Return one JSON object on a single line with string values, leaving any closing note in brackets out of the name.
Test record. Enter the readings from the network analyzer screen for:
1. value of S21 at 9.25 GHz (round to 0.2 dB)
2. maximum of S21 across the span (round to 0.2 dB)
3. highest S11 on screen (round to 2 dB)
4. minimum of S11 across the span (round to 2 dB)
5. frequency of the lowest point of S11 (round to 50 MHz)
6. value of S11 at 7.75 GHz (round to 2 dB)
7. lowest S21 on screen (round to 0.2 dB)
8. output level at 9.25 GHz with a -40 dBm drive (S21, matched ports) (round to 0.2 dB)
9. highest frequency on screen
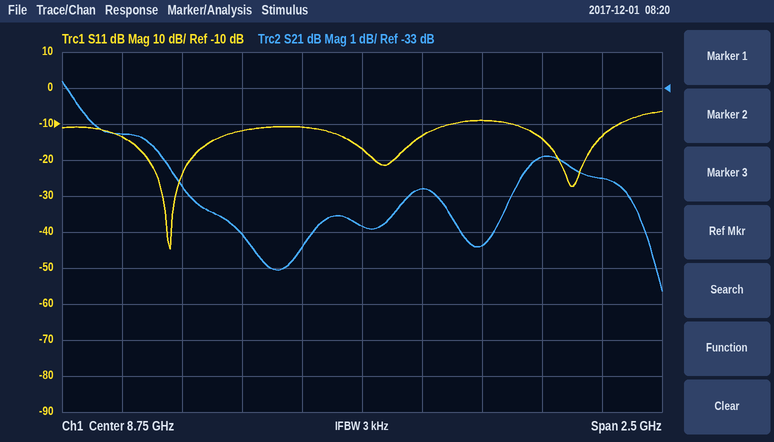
{"value of S21 at 9.25 GHz": "-37.4 dB", "maximum of S21 across the span": "-32.8 dB", "highest S11 on screen": "-6 dB", "minimum of S11 across the span": "-44 dB", "frequency of the lowest point of S11": "7.95 GHz", "value of S11 at 7.75 GHz": "-14 dB", "lowest S21 on screen": "-38.6 dB", "output level at 9.25 GHz with a -40 dBm drive (S21, matched ports)": "-77.4 dBm", "highest frequency on screen": "10 GHz"}
